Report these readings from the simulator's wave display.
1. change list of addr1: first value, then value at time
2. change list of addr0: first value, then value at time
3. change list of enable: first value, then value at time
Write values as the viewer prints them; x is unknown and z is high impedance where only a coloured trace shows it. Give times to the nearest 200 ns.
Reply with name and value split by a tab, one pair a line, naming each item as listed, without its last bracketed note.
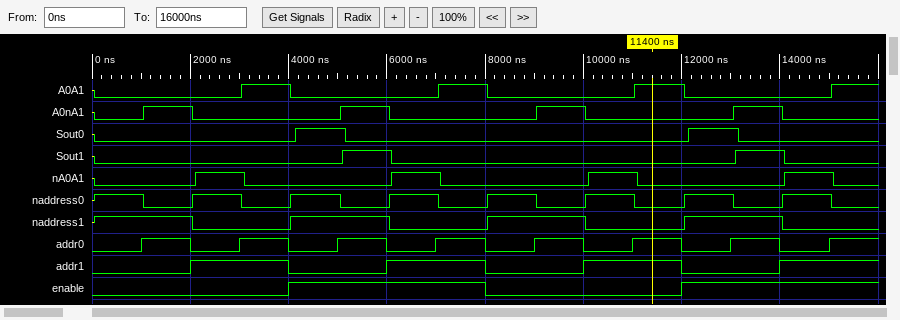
change list of addr1: first value, then value at time	0, 1 at 2000 ns, 0 at 4000 ns, 1 at 6000 ns, 0 at 8000 ns, 1 at 10000 ns, 0 at 12000 ns, 1 at 14000 ns
change list of addr0: first value, then value at time	0, 1 at 1000 ns, 0 at 2000 ns, 1 at 3000 ns, 0 at 4000 ns, 1 at 5000 ns, 0 at 6000 ns, 1 at 7000 ns, 0 at 8000 ns, 1 at 9000 ns, 0 at 10000 ns, 1 at 11000 ns, 0 at 12000 ns, 1 at 13000 ns, 0 at 14000 ns, 1 at 15000 ns
change list of enable: first value, then value at time	0, 1 at 4000 ns, 0 at 8000 ns, 1 at 12000 ns
